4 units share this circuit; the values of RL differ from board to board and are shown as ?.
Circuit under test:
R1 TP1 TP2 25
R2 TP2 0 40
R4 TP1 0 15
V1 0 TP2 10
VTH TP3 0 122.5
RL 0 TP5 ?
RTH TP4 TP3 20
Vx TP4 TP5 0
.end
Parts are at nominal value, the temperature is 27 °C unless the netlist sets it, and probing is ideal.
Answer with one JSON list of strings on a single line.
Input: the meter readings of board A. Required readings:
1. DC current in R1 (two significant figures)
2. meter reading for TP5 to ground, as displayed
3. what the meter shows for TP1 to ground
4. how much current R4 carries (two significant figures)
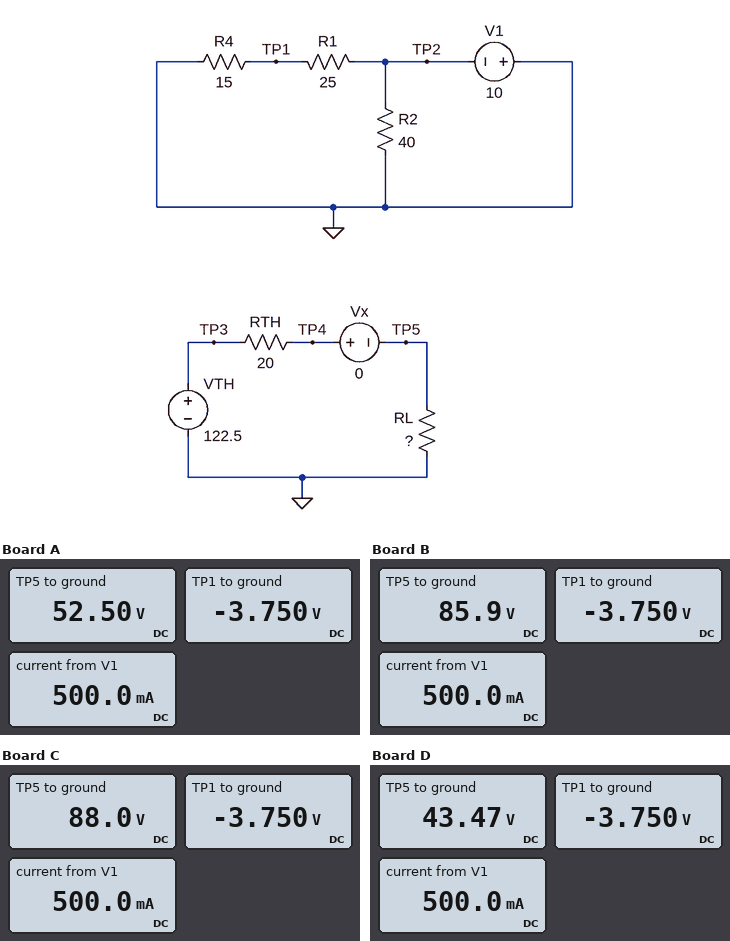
["250 mA", "52.50 V", "-3.750 V", "250 mA"]
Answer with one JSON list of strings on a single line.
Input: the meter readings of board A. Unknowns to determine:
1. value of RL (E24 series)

["15 Ω"]
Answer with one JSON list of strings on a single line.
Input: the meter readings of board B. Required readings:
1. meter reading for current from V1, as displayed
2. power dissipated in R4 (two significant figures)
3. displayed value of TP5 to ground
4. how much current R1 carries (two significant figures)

["500.0 mA", "940 mW", "85.9 V", "250 mA"]
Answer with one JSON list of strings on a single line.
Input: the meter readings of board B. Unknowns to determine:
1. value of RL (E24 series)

["47 Ω"]
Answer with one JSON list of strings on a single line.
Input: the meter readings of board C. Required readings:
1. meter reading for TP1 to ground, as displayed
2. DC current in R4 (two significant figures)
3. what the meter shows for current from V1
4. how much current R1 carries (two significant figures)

["-3.750 V", "250 mA", "500.0 mA", "250 mA"]
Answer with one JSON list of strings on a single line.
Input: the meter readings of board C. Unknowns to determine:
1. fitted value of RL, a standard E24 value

["51 Ω"]
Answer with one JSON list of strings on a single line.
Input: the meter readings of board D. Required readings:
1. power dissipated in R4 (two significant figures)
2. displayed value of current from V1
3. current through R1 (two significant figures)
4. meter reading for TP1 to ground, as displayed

["940 mW", "500.0 mA", "250 mA", "-3.750 V"]
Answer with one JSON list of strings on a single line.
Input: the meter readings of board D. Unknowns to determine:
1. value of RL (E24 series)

["11 Ω"]
